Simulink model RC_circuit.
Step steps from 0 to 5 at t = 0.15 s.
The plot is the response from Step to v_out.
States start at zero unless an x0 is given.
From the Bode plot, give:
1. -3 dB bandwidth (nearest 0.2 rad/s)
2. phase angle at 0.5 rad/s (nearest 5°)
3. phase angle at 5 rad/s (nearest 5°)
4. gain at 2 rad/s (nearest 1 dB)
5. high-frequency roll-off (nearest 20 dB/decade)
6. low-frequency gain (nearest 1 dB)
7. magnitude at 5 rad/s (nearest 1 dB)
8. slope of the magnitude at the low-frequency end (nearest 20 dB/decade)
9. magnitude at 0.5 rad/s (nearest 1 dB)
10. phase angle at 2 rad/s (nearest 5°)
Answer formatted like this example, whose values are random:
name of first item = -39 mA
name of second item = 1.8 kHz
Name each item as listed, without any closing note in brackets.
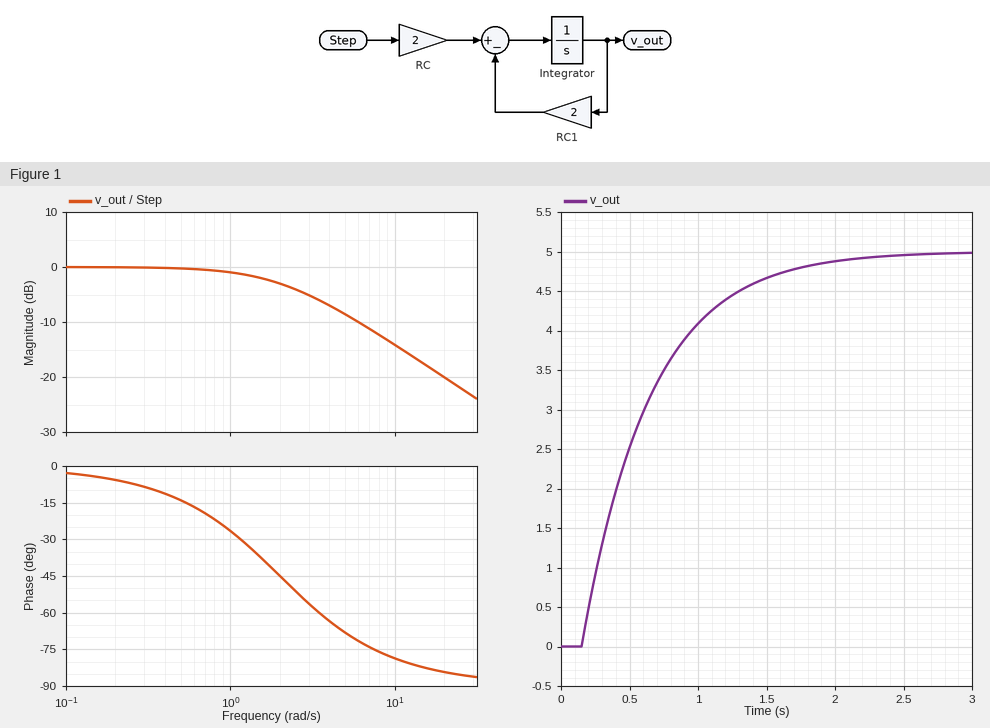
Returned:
-3 dB bandwidth = 2.0 rad/s
phase angle at 0.5 rad/s = -15°
phase angle at 5 rad/s = -70°
gain at 2 rad/s = -3 dB
high-frequency roll-off = -20 dB/decade
low-frequency gain = 0 dB
magnitude at 5 rad/s = -9 dB
slope of the magnitude at the low-frequency end = 0 dB/decade
magnitude at 0.5 rad/s = 0 dB
phase angle at 2 rad/s = -45°
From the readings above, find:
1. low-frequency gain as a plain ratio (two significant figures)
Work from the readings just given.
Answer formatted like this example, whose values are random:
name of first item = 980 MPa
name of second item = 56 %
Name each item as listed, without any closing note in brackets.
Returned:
low-frequency gain as a plain ratio = 1.0
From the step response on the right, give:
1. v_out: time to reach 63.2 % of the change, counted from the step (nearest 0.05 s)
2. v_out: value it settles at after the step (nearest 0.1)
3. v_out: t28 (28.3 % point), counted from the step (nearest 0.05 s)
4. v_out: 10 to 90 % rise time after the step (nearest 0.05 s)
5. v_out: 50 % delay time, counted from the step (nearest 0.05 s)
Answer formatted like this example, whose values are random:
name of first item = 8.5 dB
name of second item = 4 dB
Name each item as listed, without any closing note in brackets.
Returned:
v_out: time to reach 63.2 % of the change, counted from the step = 0.50 s
v_out: value it settles at after the step = 5.0
v_out: t28 (28.3 % point), counted from the step = 0.15 s
v_out: 10 to 90 % rise time after the step = 1.10 s
v_out: 50 % delay time, counted from the step = 0.35 s
